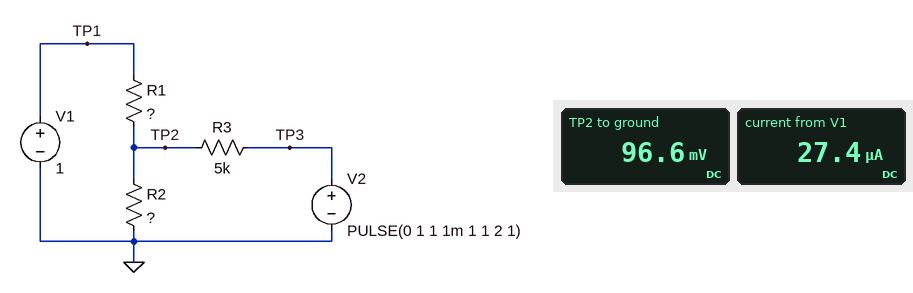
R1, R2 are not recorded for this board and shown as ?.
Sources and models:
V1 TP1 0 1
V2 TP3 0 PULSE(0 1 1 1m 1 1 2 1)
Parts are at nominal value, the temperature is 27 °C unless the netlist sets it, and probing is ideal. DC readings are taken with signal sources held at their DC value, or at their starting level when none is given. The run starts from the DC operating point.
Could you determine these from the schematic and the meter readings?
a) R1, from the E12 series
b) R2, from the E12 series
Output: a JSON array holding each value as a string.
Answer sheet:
["33 kΩ", "12 kΩ"]
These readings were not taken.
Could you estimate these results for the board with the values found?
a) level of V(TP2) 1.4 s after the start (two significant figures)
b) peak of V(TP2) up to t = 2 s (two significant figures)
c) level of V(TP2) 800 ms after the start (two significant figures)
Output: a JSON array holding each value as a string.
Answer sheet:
["730 mV", "730 mV", "97 mV"]
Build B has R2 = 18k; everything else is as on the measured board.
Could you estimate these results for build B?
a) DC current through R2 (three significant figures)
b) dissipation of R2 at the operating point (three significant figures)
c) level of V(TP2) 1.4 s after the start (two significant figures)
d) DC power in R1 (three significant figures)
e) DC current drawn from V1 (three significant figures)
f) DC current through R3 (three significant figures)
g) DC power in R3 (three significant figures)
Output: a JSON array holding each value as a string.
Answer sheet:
["5.89 µA", "624 nW", "810 mV", "24.2 µW", "27.1 µA", "21.2 µA", "2.25 µW"]
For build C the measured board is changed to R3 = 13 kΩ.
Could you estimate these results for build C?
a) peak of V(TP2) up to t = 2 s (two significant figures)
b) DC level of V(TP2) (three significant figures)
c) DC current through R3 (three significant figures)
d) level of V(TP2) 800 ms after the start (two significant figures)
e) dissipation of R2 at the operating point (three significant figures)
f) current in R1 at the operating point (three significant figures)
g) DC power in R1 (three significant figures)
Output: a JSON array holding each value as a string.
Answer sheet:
["560 mV", "159 mV", "12.2 µA", "160 mV", "2.11 µW", "25.5 µA", "21.4 µW"]
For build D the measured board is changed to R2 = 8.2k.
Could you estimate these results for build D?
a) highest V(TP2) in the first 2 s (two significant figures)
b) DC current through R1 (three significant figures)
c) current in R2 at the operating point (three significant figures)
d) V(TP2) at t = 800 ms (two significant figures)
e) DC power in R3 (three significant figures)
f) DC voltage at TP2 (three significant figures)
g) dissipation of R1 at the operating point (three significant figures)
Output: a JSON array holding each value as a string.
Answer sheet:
["650 mV", "27.7 µA", "10.5 µA", "86 mV", "1.48 µW", "86.0 mV", "25.3 µW"]
